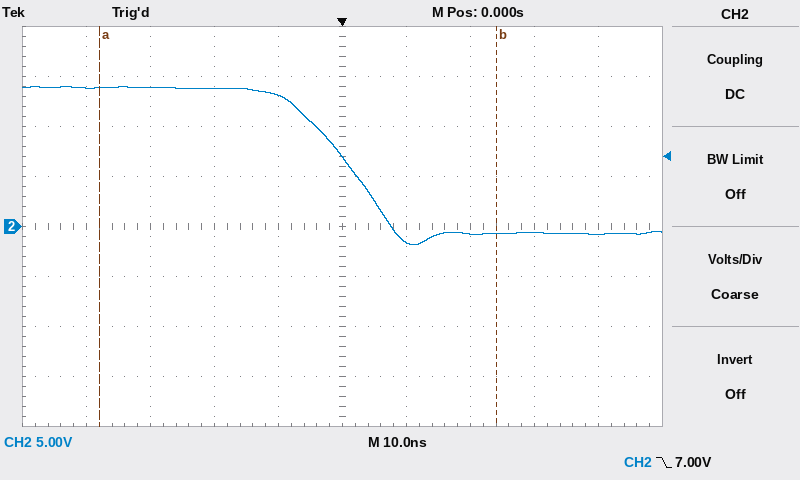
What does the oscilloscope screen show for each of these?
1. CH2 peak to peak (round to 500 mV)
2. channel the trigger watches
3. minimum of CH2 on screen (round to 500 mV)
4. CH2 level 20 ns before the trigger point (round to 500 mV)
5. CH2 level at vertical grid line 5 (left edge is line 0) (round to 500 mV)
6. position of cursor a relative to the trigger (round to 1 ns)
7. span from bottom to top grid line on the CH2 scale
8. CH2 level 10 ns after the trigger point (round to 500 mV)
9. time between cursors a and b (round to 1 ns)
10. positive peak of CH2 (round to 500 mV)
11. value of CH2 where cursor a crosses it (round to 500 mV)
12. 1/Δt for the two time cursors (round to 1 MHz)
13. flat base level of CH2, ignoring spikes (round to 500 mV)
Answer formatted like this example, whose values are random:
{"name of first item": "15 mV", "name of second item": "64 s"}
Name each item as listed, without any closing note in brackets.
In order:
{"CH2 peak to peak": "16.0 V", "channel the trigger watches": "CH2", "minimum of CH2 on screen": "-2.0 V", "CH2 level 20 ns before the trigger point": "14.0 V", "CH2 level at vertical grid line 5 (left edge is line 0)": "7.0 V", "position of cursor a relative to the trigger": "-38 ns", "span from bottom to top grid line on the CH2 scale": "40 V", "CH2 level 10 ns after the trigger point": "-1.5 V", "time between cursors a and b": "62 ns", "positive peak of CH2": "14.0 V", "value of CH2 where cursor a crosses it": "14.0 V", "1/Δt for the two time cursors": "16 MHz", "flat base level of CH2, ignoring spikes": "-500 mV"}
